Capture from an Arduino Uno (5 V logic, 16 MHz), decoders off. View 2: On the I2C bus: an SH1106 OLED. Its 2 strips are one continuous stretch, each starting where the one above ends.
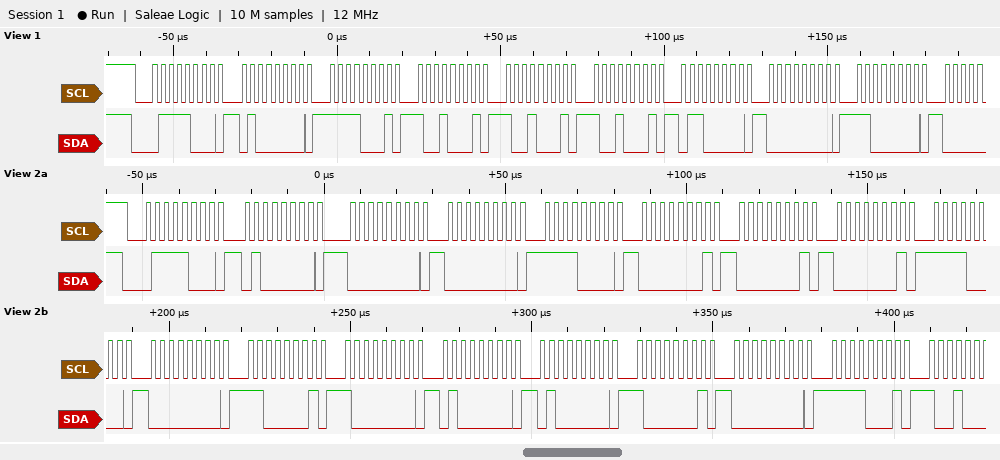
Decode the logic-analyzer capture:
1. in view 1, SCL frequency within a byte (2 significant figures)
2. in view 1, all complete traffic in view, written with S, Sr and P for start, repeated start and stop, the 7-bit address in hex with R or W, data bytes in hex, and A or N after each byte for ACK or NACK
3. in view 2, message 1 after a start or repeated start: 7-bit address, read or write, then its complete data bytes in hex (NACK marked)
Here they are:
400 kHz
S 3CW A 40 A F1 A 91 A 91 A 91 A 60 A 00 A C0 A
0x3C write: 40 00 00 F0 01 01 01 F0 00 C1 80 40 40 81 00 F1
